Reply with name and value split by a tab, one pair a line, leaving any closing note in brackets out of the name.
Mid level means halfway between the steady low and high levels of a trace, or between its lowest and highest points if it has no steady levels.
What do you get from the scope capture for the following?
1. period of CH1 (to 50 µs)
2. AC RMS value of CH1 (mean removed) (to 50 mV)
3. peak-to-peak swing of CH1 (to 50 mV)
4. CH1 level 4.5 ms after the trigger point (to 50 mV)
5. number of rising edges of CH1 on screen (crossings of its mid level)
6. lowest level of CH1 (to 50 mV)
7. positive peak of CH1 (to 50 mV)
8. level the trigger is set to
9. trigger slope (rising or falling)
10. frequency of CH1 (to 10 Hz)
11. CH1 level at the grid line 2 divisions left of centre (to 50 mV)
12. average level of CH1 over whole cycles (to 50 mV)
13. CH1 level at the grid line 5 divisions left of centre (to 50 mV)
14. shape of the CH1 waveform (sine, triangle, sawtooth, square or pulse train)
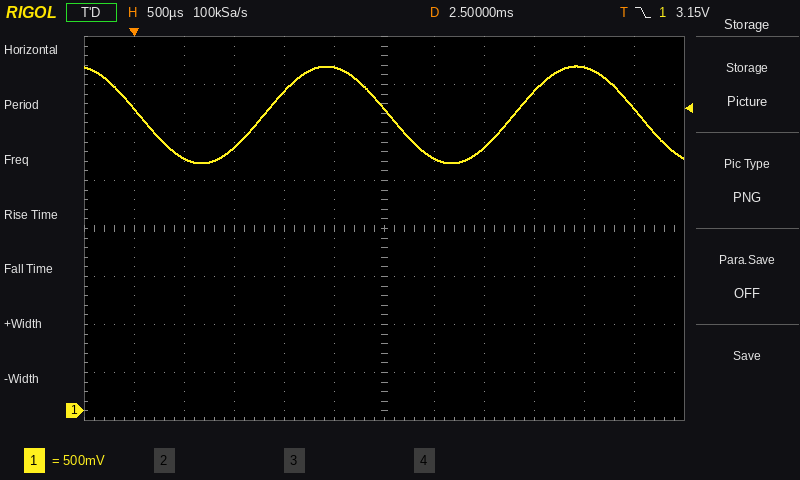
period of CH1	2.50 ms
AC RMS value of CH1 (mean removed)	350 mV
peak-to-peak swing of CH1	1.00 V
CH1 level 4.5 ms after the trigger point	3.60 V
number of rising edges of CH1 on screen	2
lowest level of CH1	2.60 V
positive peak of CH1	3.60 V
level the trigger is set to	3.15 V
trigger slope	falling
frequency of CH1	400 Hz
CH1 level at the grid line 2 divisions left of centre	3.35 V
average level of CH1 over whole cycles	3.10 V
CH1 level at the grid line 5 divisions left of centre	3.15 V
shape of the CH1 waveform	sine
